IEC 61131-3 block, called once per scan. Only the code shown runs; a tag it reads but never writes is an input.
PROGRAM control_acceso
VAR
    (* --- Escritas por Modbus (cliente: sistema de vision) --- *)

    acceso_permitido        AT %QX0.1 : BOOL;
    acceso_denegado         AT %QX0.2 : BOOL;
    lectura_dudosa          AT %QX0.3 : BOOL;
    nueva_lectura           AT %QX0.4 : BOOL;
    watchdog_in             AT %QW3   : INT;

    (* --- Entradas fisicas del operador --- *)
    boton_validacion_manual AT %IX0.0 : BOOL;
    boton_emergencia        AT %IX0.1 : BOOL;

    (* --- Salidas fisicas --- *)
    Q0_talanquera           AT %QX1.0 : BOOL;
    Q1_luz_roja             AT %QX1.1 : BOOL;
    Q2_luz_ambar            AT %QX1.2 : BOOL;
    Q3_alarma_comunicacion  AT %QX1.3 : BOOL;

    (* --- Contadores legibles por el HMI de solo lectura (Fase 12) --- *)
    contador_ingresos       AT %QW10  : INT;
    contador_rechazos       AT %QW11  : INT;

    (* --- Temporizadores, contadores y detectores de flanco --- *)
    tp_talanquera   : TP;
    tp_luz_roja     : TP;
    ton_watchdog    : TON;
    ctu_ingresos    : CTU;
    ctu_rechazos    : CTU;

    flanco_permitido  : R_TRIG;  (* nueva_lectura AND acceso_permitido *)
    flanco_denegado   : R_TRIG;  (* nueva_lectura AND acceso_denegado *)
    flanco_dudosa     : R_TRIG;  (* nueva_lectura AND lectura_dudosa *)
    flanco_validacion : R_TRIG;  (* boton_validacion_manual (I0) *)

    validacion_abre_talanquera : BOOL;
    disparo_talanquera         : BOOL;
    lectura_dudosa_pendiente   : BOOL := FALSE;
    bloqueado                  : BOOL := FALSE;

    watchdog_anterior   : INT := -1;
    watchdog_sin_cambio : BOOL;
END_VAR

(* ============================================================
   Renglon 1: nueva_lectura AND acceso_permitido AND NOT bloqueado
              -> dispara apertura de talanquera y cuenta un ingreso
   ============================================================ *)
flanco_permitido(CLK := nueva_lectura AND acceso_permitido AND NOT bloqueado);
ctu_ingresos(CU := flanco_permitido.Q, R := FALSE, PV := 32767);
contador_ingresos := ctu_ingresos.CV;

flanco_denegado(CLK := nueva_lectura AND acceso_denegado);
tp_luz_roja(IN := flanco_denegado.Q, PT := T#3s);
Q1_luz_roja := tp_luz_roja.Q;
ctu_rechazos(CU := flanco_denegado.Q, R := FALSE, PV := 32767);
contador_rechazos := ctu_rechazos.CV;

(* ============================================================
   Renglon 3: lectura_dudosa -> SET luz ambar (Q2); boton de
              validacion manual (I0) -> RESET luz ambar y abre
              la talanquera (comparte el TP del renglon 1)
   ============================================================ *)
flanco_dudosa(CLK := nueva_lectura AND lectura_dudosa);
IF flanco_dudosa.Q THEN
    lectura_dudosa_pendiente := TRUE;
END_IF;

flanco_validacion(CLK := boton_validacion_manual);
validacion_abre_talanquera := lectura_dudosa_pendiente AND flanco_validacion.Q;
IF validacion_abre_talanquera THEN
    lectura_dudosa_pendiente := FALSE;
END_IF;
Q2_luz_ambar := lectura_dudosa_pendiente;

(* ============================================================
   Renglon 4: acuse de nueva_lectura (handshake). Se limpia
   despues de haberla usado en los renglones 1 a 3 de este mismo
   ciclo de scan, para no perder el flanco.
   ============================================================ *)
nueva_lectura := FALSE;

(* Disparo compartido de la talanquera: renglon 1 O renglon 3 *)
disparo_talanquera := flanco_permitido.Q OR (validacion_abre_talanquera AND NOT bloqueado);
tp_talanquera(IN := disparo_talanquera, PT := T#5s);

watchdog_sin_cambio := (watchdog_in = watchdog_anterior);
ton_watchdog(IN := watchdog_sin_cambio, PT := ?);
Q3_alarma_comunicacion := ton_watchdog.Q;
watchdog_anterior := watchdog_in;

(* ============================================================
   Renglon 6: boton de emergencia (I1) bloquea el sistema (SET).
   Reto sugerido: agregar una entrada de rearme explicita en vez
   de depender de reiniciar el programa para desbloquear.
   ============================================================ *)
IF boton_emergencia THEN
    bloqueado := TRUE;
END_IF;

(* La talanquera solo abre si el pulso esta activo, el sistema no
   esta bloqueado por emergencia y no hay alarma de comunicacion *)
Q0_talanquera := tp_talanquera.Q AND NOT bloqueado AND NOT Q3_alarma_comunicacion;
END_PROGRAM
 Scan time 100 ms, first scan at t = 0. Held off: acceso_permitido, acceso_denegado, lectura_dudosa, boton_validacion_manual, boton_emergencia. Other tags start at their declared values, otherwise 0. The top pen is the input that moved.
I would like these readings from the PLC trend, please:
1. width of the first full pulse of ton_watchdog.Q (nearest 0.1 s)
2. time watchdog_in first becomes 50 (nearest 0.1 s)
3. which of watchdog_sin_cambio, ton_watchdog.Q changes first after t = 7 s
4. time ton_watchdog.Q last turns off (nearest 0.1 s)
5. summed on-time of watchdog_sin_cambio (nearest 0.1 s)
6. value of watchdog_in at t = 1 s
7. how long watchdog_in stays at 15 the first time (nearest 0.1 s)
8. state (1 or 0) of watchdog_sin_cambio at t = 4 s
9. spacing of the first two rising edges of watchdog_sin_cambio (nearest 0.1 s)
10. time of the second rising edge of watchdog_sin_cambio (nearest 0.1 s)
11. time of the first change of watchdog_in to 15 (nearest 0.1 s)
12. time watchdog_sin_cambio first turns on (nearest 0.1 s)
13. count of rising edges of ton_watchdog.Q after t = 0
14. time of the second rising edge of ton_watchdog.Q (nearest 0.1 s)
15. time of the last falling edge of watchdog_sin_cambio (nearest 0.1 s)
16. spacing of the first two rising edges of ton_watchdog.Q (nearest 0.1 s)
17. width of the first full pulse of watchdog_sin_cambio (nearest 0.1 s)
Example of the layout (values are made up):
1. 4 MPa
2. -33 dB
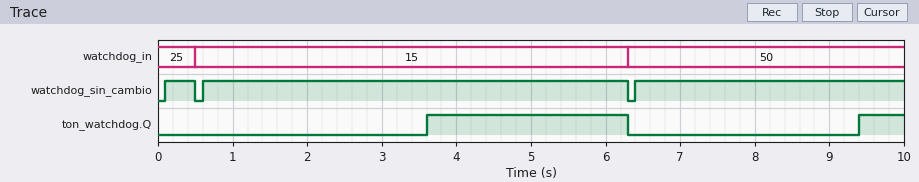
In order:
1. 2.7 s
2. 6.3 s
3. ton_watchdog.Q
4. 6.3 s
5. 9.7 s
6. 15
7. 5.8 s
8. 1
9. 0.5 s
10. 0.6 s
11. 0.5 s
12. 0.1 s
13. 2
14. 9.4 s
15. 6.3 s
16. 5.8 s
17. 0.4 s
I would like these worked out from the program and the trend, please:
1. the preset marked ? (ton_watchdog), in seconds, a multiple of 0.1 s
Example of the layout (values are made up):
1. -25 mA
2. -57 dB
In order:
1. 3.0 s
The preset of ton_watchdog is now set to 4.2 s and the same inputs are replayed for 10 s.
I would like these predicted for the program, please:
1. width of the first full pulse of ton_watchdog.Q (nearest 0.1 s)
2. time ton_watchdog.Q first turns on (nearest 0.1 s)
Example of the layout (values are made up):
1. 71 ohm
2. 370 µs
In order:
1. 1.5 s
2. 4.8 s
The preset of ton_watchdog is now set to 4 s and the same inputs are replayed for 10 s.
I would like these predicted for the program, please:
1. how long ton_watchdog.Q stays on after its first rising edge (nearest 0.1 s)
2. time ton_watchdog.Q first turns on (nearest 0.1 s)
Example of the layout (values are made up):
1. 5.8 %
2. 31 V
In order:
1. 1.7 s
2. 4.6 s
